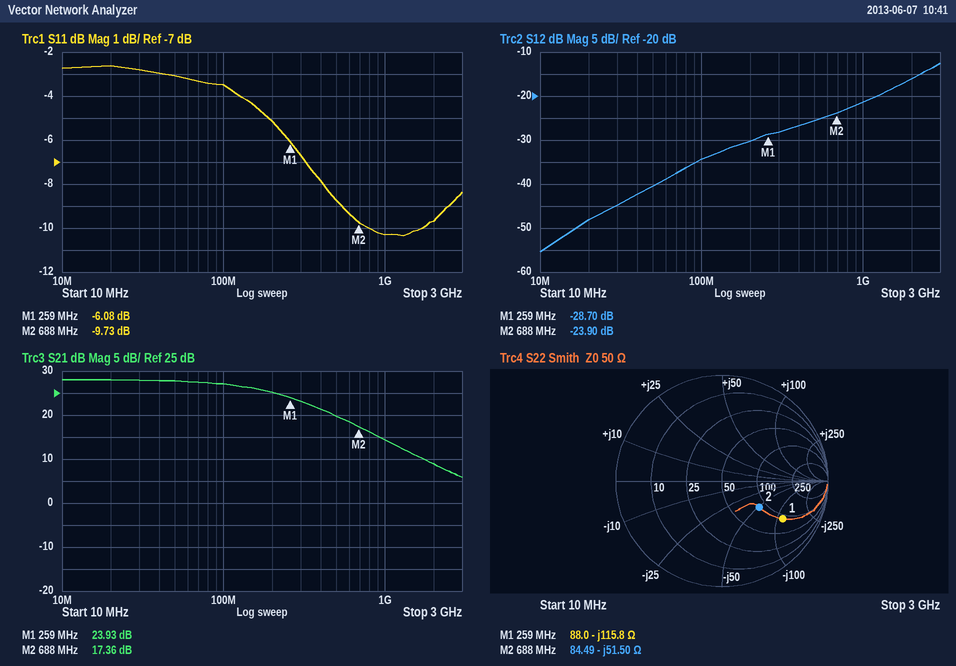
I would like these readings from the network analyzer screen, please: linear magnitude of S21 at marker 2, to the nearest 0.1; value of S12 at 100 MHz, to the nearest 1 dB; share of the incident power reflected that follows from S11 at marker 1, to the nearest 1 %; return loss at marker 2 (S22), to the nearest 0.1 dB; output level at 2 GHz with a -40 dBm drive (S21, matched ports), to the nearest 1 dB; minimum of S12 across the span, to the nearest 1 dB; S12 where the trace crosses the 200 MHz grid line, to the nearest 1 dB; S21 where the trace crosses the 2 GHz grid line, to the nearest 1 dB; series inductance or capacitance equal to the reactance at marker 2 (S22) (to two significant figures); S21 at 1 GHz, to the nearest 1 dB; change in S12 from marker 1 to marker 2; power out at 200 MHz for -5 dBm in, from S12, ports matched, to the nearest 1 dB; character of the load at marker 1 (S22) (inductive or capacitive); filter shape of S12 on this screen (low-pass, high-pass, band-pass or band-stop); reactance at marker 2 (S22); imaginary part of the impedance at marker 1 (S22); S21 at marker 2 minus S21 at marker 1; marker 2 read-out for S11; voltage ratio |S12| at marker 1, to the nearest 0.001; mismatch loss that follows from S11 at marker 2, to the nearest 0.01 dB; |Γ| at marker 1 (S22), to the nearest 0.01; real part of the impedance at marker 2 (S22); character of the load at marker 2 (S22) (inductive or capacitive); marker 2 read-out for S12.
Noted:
7.4
-34 dB
25 %
7.3 dB
-31 dBm
-55 dB
-30 dB
9 dB
4.5 pF
14 dB
4.80 dB
-35 dBm
capacitive
high-pass
-51.50 Ω
-115.8 Ω
-6.57 dB
-9.73 dB
0.037
0.49 dB
0.68
84.49 Ω
capacitive
-23.90 dB
